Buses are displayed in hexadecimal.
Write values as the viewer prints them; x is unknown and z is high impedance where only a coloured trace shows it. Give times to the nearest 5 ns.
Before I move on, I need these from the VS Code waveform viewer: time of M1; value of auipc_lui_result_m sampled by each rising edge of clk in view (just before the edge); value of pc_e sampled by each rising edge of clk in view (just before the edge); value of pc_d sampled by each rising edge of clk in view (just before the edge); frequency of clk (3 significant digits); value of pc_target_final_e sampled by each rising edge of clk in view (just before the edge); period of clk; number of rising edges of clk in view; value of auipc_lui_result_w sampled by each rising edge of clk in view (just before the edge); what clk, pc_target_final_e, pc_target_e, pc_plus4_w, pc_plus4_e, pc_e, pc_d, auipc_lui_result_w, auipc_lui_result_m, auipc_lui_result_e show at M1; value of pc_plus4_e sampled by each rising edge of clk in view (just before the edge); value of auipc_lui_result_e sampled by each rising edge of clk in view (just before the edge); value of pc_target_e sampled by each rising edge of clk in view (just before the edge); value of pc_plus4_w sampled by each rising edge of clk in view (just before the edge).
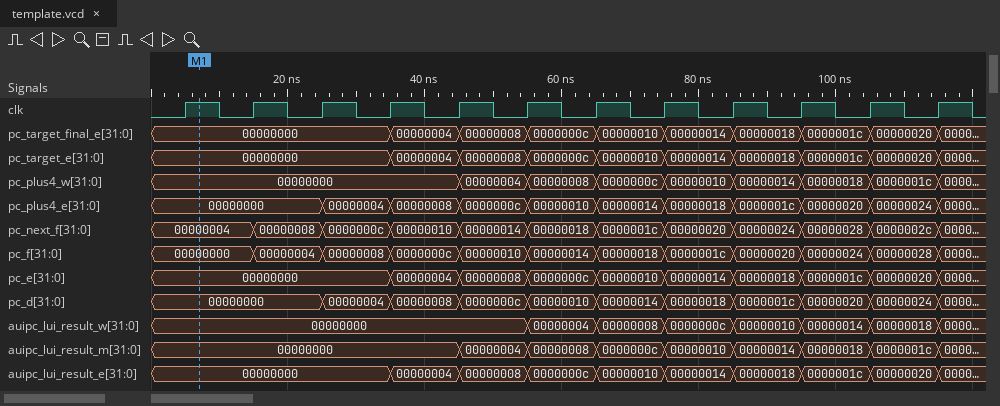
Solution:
5 ns
00000000, 00000000, 00000000, 00000000, 00000000, 00000004, 00000008, 0000000c, 00000010, 00000014, 00000018, 0000001c
00000000, 00000000, 00000000, 00000000, 00000004, 00000008, 0000000c, 00000010, 00000014, 00000018, 0000001c, 00000020
00000000, 00000000, 00000000, 00000004, 00000008, 0000000c, 00000010, 00000014, 00000018, 0000001c, 00000020, 00000024
100 MHz
00000000, 00000000, 00000000, 00000000, 00000004, 00000008, 0000000c, 00000010, 00000014, 00000018, 0000001c, 00000020
10 ns
12
00000000, 00000000, 00000000, 00000000, 00000000, 00000000, 00000004, 00000008, 0000000c, 00000010, 00000014, 00000018
clk=1, pc_target_final_e=00000000, pc_target_e=00000000, pc_plus4_w=00000000, pc_plus4_e=00000000, pc_e=00000000, pc_d=00000000, auipc_lui_result_w=00000000, auipc_lui_result_m=00000000, auipc_lui_result_e=00000000
00000000, 00000000, 00000000, 00000004, 00000008, 0000000c, 00000010, 00000014, 00000018, 0000001c, 00000020, 00000024
00000000, 00000000, 00000000, 00000000, 00000004, 00000008, 0000000c, 00000010, 00000014, 00000018, 0000001c, 00000020
00000000, 00000000, 00000000, 00000000, 00000004, 00000008, 0000000c, 00000010, 00000014, 00000018, 0000001c, 00000020
00000000, 00000000, 00000000, 00000000, 00000000, 00000004, 00000008, 0000000c, 00000010, 00000014, 00000018, 0000001c
